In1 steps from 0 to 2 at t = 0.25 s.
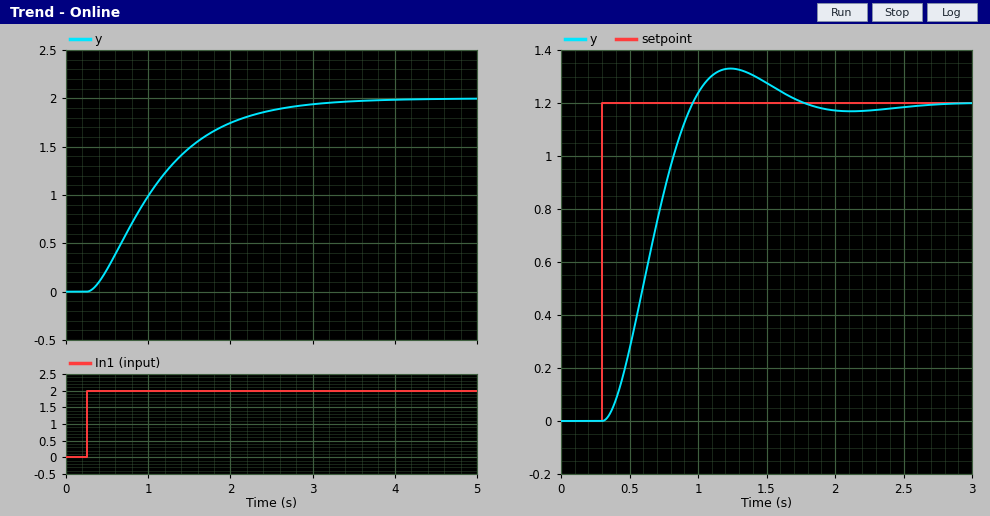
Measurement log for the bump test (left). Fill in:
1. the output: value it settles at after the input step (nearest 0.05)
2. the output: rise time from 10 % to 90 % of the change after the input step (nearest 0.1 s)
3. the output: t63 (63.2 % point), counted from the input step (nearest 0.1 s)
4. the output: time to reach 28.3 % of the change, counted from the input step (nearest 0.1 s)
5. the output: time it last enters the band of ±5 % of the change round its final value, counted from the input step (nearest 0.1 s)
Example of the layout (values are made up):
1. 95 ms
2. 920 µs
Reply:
1. 2.00
2. 1.7 s
3. 1.0 s
4. 0.5 s
5. 2.4 s
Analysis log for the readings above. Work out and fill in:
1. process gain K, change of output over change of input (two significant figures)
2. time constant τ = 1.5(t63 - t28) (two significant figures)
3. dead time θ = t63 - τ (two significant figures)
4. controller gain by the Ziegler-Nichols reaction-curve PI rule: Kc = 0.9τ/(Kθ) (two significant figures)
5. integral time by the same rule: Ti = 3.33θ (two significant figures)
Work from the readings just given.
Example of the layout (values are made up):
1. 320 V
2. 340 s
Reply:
1. 1.0
2. 0.75 s
3. 0.25 s
4. 2.7
5. 0.83 s
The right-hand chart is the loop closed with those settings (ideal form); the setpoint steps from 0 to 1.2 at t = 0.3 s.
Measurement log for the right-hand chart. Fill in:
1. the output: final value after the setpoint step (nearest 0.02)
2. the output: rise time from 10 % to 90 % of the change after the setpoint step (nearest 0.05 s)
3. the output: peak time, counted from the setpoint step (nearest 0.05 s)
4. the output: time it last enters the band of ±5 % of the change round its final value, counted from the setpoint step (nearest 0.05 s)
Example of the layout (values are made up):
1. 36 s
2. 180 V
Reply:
1. 1.20
2. 0.45 s
3. 0.95 s
4. 1.25 s
